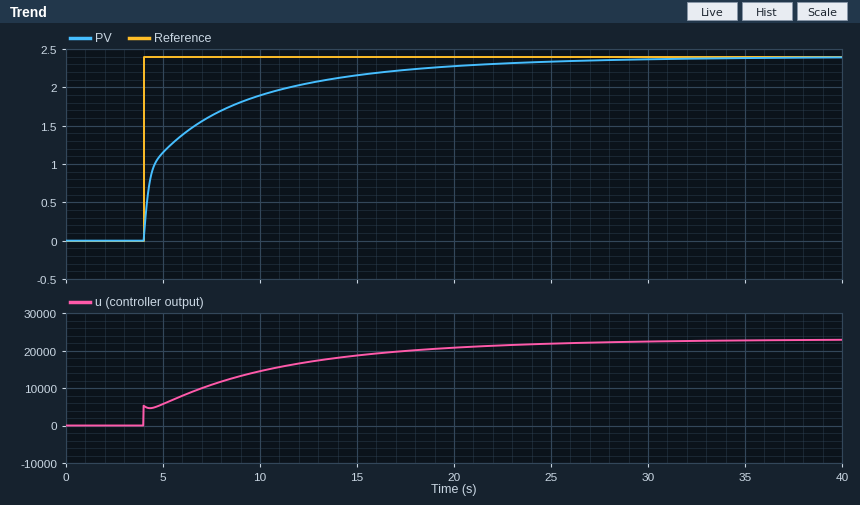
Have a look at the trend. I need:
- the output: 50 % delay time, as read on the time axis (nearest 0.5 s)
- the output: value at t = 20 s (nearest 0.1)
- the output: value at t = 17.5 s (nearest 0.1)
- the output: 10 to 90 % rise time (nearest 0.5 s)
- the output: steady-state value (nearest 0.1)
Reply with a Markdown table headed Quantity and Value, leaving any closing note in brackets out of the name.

| Quantity | Value |
|---|---|
| the output: 50 % delay time, as read on the time axis | 5.0 s |
| the output: value at t = 20 s | 2.3 |
| the output: value at t = 17.5 s | 2.2 |
| the output: 10 to 90 % rise time | 11.0 s |
| the output: steady-state value | 2.4 |
